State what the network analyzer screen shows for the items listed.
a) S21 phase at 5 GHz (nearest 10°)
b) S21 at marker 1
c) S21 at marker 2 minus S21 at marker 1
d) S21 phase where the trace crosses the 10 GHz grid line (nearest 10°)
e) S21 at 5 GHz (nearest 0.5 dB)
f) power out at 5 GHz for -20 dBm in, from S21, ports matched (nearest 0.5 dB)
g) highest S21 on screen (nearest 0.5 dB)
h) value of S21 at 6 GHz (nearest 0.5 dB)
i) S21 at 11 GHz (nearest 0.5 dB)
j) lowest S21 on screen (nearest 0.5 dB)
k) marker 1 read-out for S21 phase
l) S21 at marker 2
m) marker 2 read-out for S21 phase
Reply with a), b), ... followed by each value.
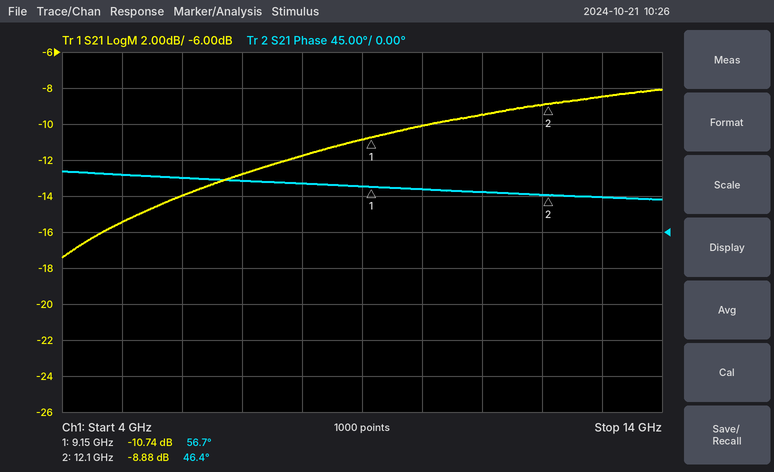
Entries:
a) 70°
b) -10.74 dB
c) 1.86 dB
d) 50°
e) -15.5 dB
f) -35.5 dBm
g) -8.0 dB
h) -14.0 dB
i) -9.5 dB
j) -17.5 dB
k) 56.7°
l) -8.88 dB
m) 46.4°
